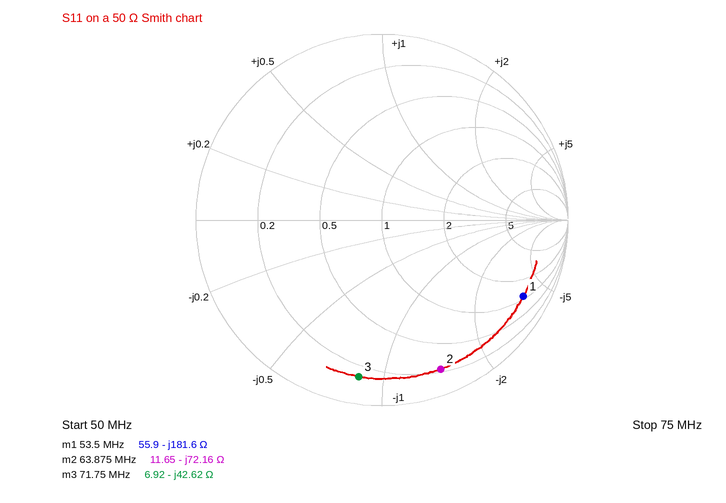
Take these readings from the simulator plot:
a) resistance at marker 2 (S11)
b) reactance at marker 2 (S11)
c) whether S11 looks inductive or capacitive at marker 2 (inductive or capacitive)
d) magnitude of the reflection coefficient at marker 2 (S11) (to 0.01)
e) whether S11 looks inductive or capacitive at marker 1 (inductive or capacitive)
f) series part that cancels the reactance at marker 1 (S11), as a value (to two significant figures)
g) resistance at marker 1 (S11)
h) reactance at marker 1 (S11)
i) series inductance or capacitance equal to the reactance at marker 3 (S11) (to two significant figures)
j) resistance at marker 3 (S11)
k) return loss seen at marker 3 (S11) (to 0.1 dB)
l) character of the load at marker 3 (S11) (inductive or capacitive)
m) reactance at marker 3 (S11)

11.65 Ω
-72.16 Ω
capacitive
0.86
capacitive
540 nH
55.9 Ω
-181.6 Ω
52 pF
6.92 Ω
1.4 dB
capacitive
-42.62 Ω
